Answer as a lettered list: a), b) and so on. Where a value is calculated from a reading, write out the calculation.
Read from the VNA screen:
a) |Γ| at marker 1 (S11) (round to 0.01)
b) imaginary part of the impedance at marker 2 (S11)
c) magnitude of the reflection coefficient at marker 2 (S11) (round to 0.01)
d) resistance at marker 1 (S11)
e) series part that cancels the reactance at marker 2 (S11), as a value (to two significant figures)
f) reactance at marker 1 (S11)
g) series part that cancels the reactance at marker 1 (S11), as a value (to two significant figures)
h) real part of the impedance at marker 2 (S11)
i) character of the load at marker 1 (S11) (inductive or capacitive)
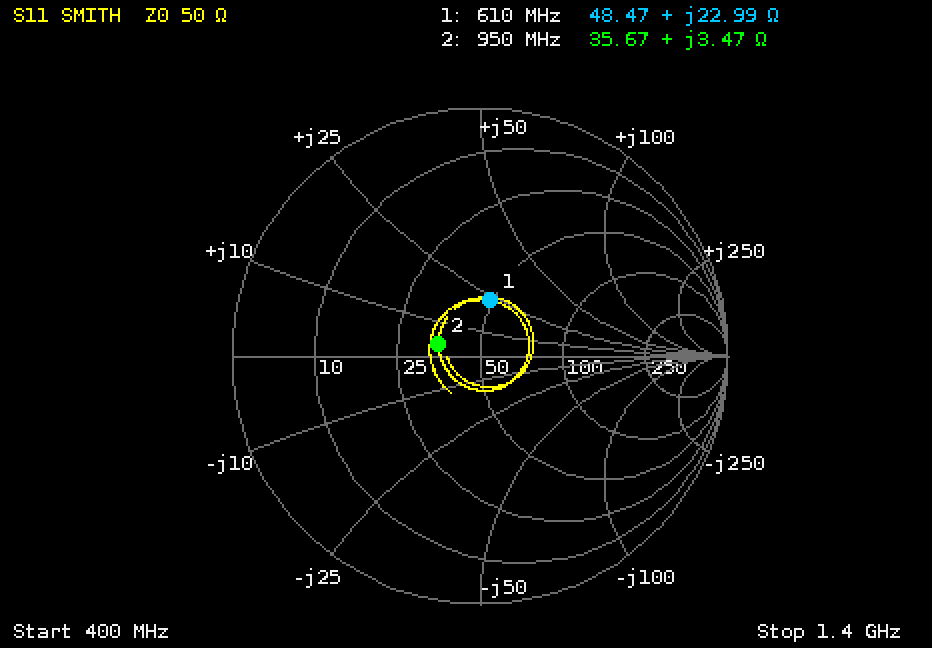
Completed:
a) 0.23
b) +3.47 Ω
c) 0.17
d) 48.47 Ω
e) C = 1/(2π × 950 MHz × 3.47 Ω) ≈ 48 pF
f) +22.99 Ω
g) C = 1/(2π × 610 MHz × 22.99 Ω) ≈ 11 pF
h) 35.67 Ω
i) inductive
